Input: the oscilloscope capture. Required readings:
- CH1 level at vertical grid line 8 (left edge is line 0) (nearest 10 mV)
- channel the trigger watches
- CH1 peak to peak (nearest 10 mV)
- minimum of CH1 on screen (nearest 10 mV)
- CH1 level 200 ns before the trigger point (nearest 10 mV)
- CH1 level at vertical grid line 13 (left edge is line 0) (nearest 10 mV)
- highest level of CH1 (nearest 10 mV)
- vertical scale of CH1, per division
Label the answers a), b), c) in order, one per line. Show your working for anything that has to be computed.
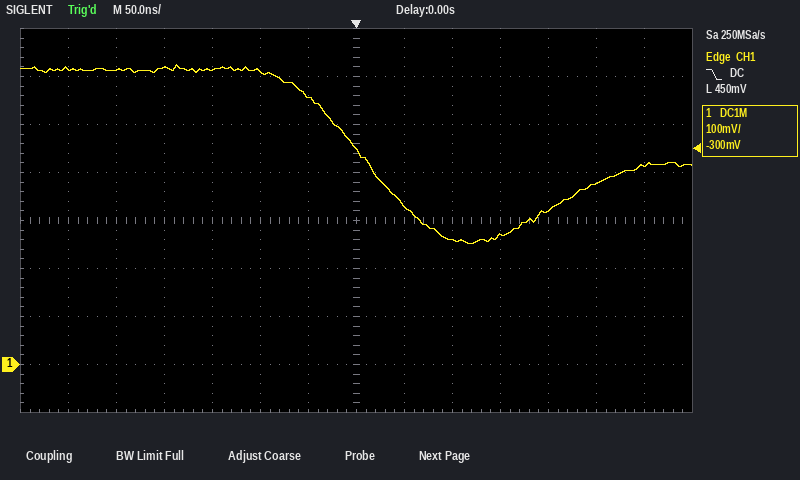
a) 330 mV
b) CH1
c) 620 mV − (250 mV) = 370 mV
d) 250 mV
e) 620 mV
f) 410 mV
g) 620 mV
h) 100 mV
